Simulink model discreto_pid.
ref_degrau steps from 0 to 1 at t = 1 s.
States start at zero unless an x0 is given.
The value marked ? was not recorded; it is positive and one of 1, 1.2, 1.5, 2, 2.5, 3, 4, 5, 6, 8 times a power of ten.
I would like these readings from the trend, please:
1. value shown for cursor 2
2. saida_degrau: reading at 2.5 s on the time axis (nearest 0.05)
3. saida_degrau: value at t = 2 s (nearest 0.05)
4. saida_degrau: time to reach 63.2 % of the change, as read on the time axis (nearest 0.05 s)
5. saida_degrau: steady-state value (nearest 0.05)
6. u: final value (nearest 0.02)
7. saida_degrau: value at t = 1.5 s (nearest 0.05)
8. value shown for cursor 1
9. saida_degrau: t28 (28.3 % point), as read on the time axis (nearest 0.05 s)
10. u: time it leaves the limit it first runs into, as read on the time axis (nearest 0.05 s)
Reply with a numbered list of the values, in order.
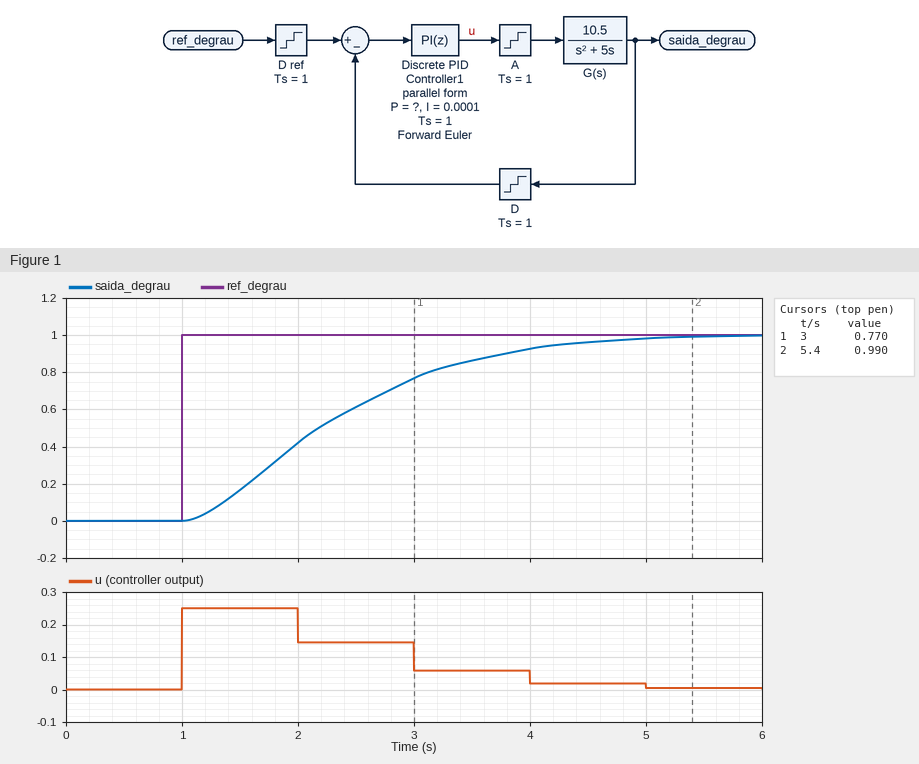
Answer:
1. 0.990
2. 0.60
3. 0.40
4. 2.55 s
5. 1.00
6. 0.00
7. 0.15
8. 0.770
9. 1.75 s
10. 2.00 s
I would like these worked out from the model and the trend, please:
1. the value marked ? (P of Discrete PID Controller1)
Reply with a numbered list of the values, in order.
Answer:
1. 0.25
